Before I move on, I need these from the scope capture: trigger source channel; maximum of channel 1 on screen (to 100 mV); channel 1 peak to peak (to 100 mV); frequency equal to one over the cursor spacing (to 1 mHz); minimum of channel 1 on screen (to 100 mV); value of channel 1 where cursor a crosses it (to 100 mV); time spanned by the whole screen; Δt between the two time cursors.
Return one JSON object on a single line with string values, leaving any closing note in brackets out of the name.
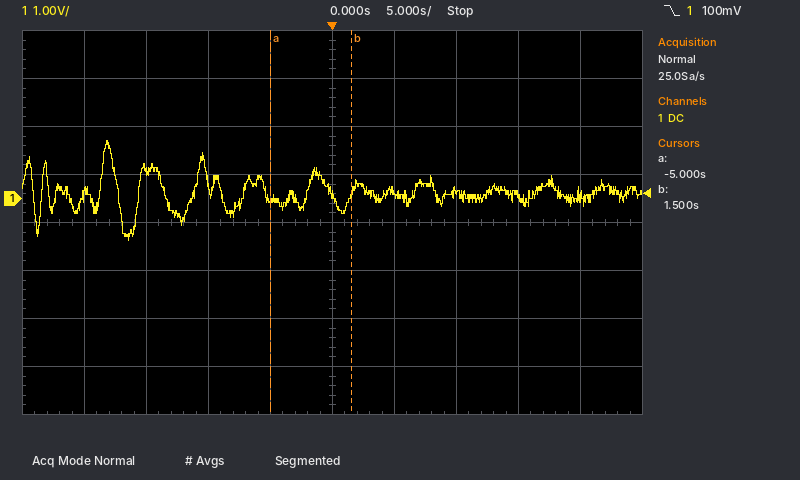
{"trigger source channel": "channel 1", "maximum of channel 1 on screen": "1.2 V", "channel 1 peak to peak": "2.1 V", "frequency equal to one over the cursor spacing": "154 mHz", "minimum of channel 1 on screen": "-900 mV", "value of channel 1 where cursor a crosses it": "0.0 V", "time spanned by the whole screen": "50 s", "Δt between the two time cursors": "6.5 s"}
